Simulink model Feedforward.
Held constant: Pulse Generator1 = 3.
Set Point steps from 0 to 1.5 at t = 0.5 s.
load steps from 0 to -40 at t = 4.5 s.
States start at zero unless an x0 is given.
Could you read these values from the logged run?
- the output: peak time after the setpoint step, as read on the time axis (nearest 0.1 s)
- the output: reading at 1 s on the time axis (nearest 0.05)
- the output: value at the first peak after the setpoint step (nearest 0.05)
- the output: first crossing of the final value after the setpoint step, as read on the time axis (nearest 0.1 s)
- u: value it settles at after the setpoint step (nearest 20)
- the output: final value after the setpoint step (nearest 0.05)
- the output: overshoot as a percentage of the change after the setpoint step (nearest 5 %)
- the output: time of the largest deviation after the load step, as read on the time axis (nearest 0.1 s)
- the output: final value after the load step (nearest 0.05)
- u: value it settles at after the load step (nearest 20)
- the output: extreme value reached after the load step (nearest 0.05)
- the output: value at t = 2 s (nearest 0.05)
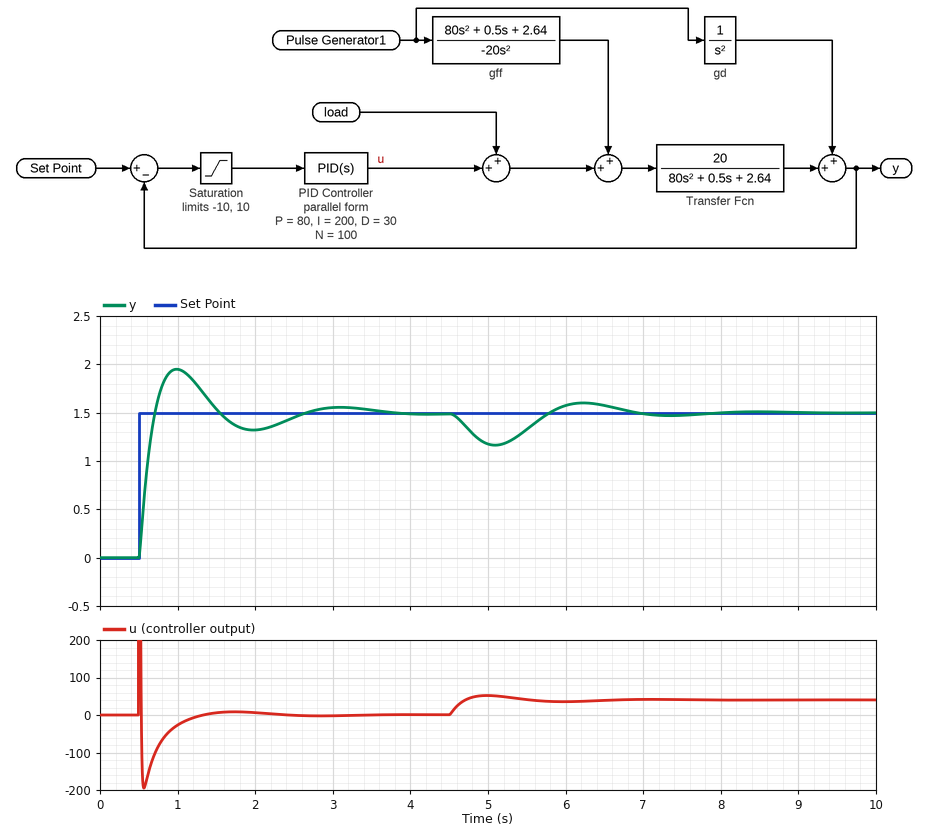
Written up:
1.0 s
1.95
1.95
0.7 s
0
1.50
30 %
5.1 s
1.50
40
1.15
1.30
